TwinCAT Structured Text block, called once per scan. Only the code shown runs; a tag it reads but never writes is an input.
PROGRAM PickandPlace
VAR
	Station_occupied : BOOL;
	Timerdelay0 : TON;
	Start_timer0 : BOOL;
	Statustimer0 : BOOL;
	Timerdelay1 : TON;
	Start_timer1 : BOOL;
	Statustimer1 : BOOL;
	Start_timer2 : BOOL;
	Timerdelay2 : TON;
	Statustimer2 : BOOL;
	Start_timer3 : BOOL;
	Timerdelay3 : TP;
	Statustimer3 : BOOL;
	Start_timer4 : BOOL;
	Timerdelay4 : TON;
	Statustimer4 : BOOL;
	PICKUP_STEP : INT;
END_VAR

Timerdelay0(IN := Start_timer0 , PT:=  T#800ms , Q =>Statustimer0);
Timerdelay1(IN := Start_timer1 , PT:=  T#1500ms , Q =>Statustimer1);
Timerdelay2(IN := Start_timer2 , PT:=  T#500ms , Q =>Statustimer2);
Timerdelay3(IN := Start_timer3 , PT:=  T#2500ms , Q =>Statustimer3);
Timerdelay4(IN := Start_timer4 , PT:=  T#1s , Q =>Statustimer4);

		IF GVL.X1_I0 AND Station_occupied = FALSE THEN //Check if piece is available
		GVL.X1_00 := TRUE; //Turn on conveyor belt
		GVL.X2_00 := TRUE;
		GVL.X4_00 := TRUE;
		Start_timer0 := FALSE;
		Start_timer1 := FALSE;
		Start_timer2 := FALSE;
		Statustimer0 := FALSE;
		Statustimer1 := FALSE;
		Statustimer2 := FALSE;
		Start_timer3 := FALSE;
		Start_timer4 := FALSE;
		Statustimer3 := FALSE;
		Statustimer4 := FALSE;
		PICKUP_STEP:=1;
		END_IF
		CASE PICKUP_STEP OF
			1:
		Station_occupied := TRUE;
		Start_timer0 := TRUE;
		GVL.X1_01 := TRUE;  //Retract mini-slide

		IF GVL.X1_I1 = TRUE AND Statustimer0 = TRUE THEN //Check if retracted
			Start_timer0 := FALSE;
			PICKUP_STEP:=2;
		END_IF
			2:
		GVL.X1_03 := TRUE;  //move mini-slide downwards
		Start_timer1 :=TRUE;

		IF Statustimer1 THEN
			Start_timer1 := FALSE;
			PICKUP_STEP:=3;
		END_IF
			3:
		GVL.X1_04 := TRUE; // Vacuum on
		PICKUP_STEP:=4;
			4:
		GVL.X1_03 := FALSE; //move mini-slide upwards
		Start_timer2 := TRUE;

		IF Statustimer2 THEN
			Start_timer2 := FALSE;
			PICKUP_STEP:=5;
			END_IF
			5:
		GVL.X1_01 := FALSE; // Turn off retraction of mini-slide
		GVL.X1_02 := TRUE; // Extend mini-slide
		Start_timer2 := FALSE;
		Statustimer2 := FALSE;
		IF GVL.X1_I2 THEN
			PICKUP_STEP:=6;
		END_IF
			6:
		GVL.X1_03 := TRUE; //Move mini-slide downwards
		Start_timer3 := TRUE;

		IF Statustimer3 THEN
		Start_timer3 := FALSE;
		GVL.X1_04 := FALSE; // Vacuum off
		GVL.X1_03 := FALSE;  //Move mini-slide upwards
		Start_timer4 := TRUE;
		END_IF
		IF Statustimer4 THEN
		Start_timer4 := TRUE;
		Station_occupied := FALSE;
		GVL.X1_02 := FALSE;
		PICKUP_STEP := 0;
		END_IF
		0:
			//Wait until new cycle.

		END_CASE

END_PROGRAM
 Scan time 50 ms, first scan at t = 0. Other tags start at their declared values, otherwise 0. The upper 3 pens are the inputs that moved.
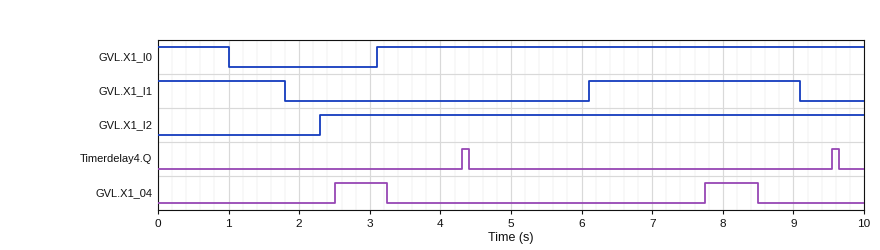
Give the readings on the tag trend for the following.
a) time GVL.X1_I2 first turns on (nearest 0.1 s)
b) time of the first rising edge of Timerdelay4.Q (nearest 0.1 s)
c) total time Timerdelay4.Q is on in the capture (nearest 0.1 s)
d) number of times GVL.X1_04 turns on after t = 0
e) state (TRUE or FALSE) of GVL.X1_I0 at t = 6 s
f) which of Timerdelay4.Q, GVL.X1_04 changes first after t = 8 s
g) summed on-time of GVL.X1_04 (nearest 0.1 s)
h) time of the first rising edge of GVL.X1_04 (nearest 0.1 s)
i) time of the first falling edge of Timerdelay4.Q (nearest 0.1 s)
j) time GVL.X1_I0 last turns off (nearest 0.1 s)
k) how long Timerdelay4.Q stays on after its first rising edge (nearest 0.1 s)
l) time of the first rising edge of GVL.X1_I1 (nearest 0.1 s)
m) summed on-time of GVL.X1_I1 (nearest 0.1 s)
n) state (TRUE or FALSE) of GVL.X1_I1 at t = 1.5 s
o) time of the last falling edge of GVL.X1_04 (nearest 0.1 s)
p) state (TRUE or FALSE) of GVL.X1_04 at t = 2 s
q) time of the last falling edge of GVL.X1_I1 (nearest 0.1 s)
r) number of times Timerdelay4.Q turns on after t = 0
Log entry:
2.3 s
4.3 s
0.2 s
2
TRUE
GVL.X1_04
1.5 s
2.5 s
4.4 s
1.0 s
0.1 s
6.1 s
4.8 s
TRUE
8.5 s
FALSE
9.1 s
2
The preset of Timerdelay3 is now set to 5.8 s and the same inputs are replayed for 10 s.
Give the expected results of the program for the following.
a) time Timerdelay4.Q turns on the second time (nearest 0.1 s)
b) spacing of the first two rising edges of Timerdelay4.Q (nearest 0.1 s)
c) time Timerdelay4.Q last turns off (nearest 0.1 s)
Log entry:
9.5 s
5.2 s
9.6 s
